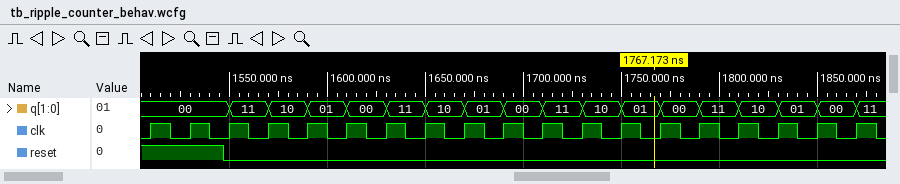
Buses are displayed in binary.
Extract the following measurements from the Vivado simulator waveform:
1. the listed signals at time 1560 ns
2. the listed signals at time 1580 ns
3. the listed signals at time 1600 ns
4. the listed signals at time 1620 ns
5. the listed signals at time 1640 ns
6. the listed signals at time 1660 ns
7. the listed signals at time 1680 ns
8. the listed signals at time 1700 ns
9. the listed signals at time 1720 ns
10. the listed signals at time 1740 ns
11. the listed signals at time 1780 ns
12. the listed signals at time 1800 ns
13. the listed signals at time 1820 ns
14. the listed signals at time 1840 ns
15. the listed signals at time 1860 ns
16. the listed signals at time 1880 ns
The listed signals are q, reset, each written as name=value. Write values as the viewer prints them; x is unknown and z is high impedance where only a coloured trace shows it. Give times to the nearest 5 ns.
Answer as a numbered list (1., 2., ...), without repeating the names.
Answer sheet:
1. q=11, reset=0
2. q=10, reset=0
3. q=01, reset=0
4. q=00, reset=0
5. q=11, reset=0
6. q=10, reset=0
7. q=01, reset=0
8. q=00, reset=0
9. q=11, reset=0
10. q=10, reset=0
11. q=00, reset=0
12. q=11, reset=0
13. q=10, reset=0
14. q=01, reset=0
15. q=00, reset=0
16. q=11, reset=0
